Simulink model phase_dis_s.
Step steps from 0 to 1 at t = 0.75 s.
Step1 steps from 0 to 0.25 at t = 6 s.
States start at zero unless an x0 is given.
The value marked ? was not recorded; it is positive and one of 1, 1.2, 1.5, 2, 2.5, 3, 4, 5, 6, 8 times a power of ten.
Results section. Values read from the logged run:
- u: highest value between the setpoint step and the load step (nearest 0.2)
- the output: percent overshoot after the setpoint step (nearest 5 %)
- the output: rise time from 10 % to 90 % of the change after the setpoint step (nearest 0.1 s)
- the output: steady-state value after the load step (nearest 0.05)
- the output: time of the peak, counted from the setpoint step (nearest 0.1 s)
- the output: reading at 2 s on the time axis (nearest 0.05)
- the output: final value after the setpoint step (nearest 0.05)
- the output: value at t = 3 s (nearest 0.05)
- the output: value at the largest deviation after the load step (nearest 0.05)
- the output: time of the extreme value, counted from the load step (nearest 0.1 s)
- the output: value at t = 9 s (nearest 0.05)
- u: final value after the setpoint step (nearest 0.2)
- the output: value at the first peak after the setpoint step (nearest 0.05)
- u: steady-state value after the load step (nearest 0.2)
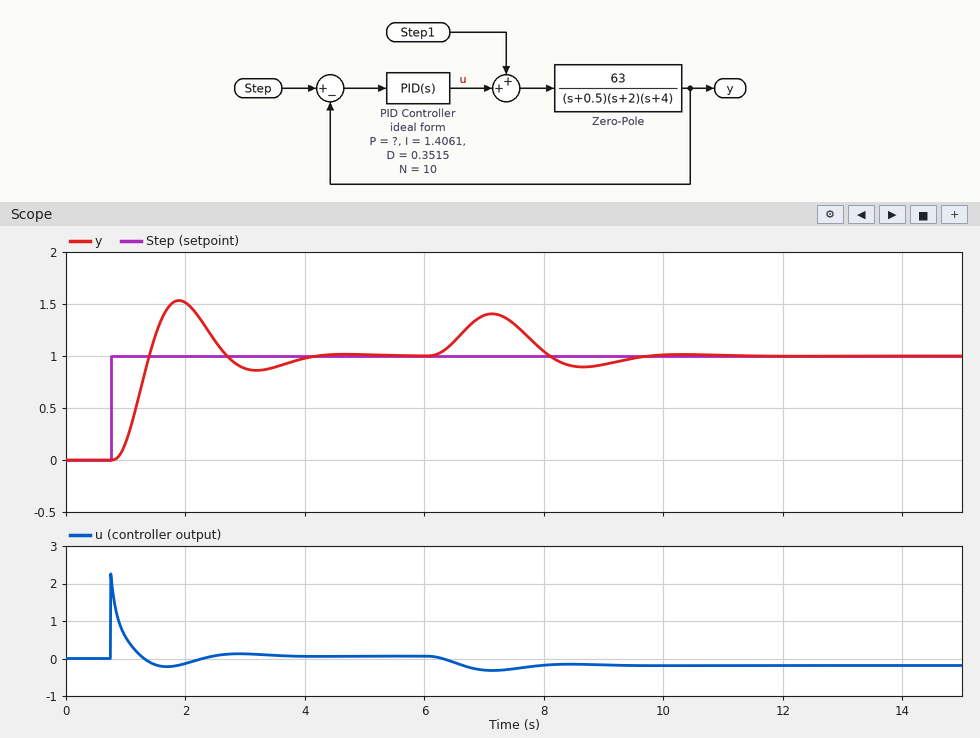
2.2
55 %
0.4 s
1.00
1.1 s
1.50
1.00
0.90
1.40
1.1 s
0.90
0.0
1.55
-0.2
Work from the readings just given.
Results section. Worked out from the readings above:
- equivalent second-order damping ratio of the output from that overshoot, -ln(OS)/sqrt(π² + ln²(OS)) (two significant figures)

0.19
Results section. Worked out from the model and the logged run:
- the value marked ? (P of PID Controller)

0.5
